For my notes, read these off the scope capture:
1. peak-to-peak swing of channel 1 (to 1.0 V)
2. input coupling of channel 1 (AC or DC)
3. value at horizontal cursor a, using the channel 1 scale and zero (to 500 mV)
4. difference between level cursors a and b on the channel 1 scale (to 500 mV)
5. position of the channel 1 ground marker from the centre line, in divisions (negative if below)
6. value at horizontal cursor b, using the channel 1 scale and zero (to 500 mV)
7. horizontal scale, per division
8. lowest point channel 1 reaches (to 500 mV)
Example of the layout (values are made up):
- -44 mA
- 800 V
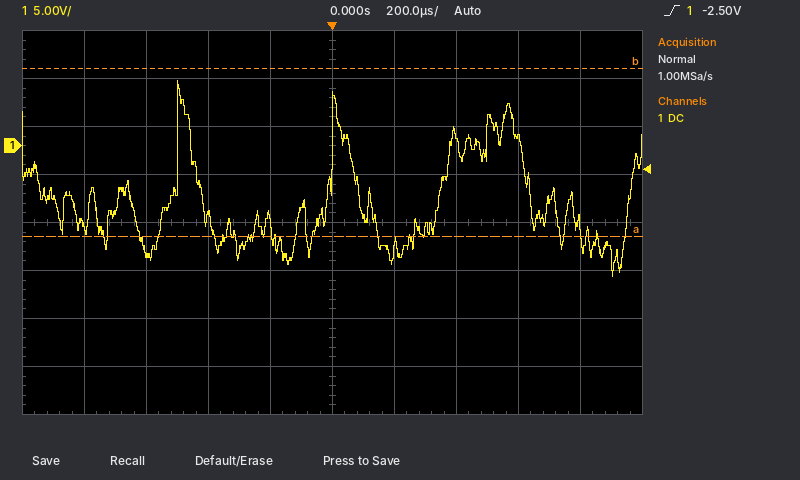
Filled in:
- 20.0 V
- DC
- -9.5 V
- 17.5 V
- +1.6 div
- 8.0 V
- 200 µs
- -13.5 V
